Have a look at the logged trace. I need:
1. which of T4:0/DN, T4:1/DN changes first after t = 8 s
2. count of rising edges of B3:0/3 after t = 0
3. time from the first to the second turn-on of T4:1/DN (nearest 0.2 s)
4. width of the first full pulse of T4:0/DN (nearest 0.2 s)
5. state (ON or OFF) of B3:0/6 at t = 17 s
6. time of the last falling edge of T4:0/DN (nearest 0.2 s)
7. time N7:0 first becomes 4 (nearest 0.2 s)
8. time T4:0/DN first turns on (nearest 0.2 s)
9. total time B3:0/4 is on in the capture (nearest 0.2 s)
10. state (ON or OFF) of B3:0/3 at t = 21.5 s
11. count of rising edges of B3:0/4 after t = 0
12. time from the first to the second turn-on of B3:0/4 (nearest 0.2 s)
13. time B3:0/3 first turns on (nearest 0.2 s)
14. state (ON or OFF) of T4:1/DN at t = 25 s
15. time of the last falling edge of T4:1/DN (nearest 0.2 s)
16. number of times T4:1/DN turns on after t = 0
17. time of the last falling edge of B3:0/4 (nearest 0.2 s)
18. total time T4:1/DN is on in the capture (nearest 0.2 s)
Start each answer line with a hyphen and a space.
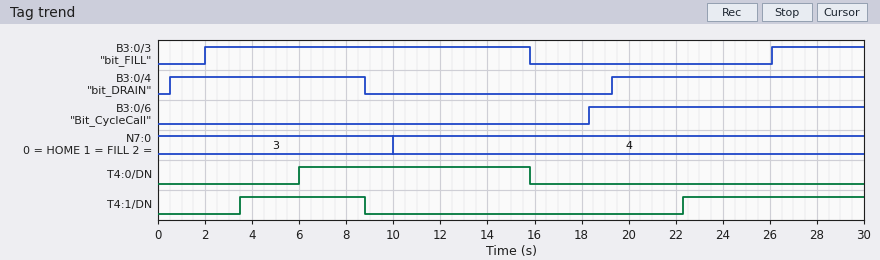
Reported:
- T4:1/DN
- 2
- 18.8 s
- 9.8 s
- OFF
- 15.8 s
- 10.0 s
- 6.0 s
- 19.0 s
- OFF
- 2
- 18.8 s
- 2.0 s
- ON
- 8.8 s
- 2
- 8.8 s
- 13.0 s
